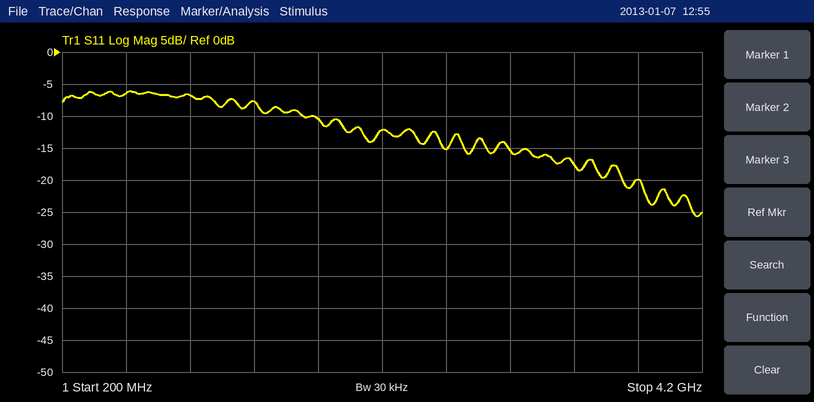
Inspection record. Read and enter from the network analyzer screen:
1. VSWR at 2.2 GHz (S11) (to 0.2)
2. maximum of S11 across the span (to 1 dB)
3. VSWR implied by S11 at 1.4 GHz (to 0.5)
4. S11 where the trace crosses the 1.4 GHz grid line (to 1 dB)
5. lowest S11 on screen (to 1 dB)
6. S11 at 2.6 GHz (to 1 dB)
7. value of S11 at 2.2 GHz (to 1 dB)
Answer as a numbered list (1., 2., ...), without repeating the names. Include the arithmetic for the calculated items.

1. |Γ| = 10^(-12/20) = 0.2512; VSWR = (1 + 0.2512)/(1 − 0.2512) ≈ 1.67, so 1.6 to the nearest 0.2
2. -6 dB
3. |Γ| = 10^(-8/20) = 0.3981; VSWR = (1 + 0.3981)/(1 − 0.3981) ≈ 2.32, so 2.5 to the nearest 0.5
4. -8 dB
5. -26 dB
6. -15 dB
7. -12 dB
